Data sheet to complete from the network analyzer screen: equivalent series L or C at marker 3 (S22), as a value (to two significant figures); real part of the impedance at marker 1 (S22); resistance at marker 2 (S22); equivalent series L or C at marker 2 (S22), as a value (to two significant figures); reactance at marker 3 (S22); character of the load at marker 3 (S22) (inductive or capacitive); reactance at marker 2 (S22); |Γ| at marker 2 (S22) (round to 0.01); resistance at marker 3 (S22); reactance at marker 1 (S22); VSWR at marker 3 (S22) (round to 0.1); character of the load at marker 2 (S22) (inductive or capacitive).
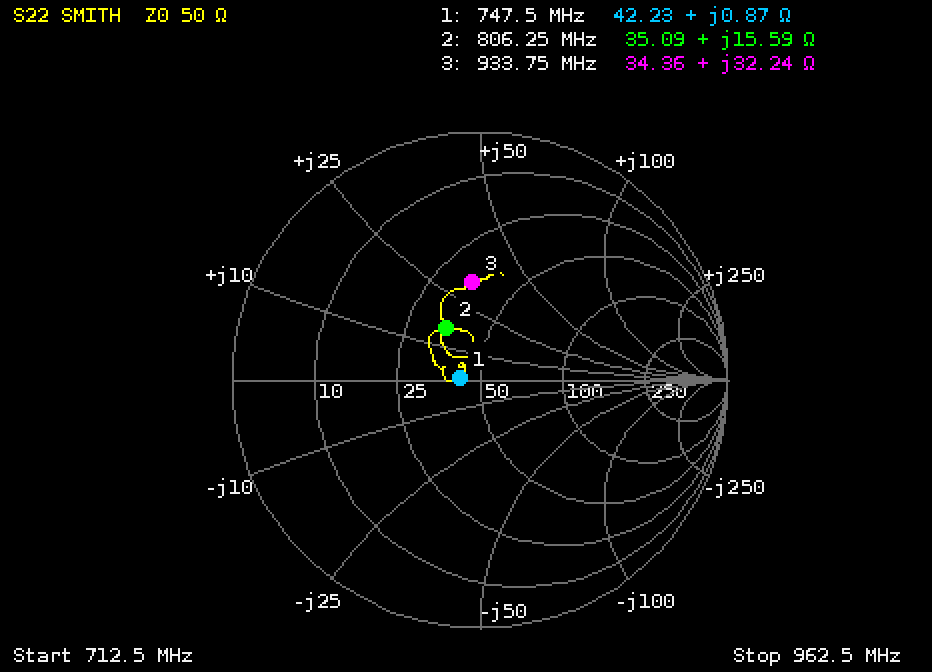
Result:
5.5 nH
42.23 Ω
35.09 Ω
3.1 nH
+32.24 Ω
inductive
+15.59 Ω
0.25
34.36 Ω
+0.87 Ω
2.3
inductive
